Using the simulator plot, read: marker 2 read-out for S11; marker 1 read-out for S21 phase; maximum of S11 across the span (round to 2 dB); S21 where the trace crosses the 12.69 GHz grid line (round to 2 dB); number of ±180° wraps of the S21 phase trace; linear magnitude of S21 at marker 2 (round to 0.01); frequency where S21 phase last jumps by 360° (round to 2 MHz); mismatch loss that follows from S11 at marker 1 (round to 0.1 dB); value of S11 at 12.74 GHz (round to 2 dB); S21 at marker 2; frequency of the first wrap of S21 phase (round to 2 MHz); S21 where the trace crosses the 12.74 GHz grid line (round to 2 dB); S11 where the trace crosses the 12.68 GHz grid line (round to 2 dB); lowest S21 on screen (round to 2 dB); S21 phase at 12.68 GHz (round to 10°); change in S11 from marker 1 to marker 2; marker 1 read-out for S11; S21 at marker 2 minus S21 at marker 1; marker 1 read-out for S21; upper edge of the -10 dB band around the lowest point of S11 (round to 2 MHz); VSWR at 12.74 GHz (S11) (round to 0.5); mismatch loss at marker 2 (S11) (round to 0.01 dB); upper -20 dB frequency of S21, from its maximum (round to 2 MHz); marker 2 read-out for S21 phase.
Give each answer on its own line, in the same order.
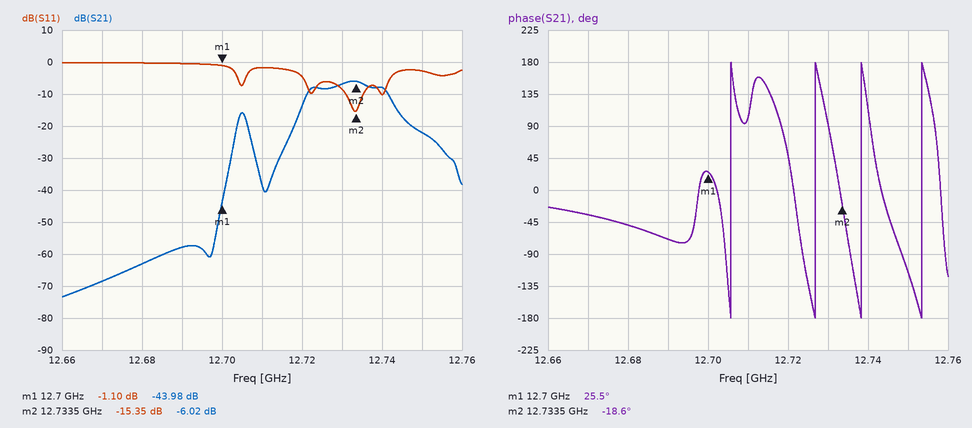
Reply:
-15.35 dB
25.5°
0 dB
-58 dB
4
0.50
12.754 GHz
6.5 dB
-10 dB
-6.02 dB
12.706 GHz
-8 dB
0 dB
-74 dB
-50°
-14.25 dB
-1.10 dB
37.96 dB
-43.98 dB
12.736 GHz
2.0
0.13 dB
12.754 GHz
-18.6°
